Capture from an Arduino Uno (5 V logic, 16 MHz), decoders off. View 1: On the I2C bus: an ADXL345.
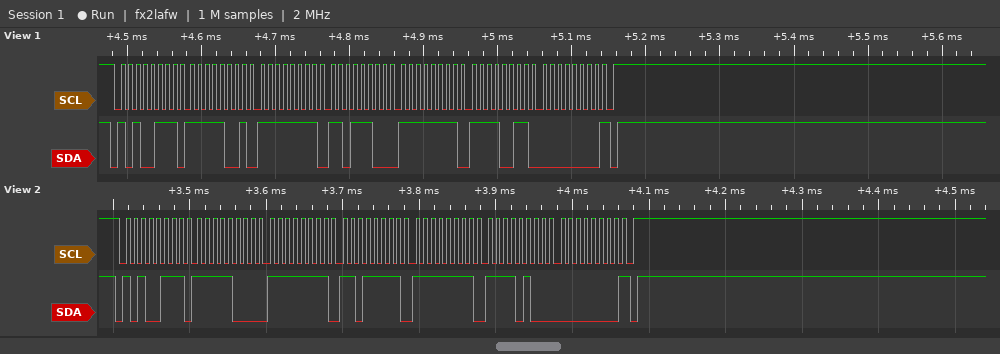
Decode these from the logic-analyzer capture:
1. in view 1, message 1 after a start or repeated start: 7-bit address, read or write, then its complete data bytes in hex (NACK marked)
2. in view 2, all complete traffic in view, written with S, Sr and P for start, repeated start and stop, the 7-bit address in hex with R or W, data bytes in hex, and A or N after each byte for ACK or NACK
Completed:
0x53 read: F9 FF DC FF F3 00 NACK
S 53R A F8 A FF A DF A FF A F4 A 00 N P
